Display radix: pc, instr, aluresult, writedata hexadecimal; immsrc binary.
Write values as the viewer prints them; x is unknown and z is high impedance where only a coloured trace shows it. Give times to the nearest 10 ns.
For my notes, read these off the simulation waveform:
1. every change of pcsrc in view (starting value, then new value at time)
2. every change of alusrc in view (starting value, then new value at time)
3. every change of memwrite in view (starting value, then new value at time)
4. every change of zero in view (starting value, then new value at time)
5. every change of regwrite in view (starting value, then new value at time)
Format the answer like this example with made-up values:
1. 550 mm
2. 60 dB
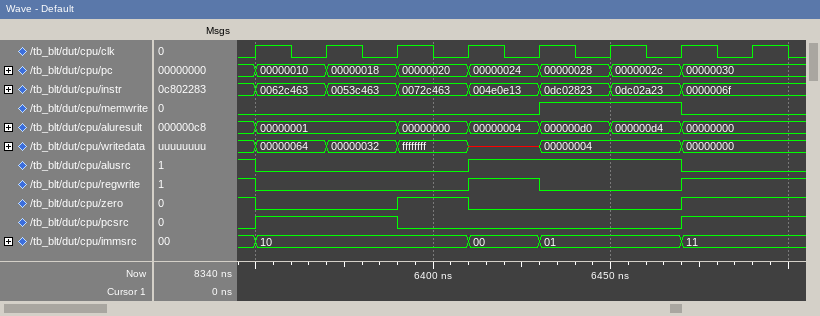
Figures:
1. 0, 1 at 6350 ns, 0 at 6390 ns, 1 at 6470 ns
2. 1, 0 at 6350 ns, 1 at 6410 ns, 0 at 6470 ns
3. 0, 1 at 6430 ns, 0 at 6470 ns
4. 1, 0 at 6350 ns, 1 at 6390 ns, 0 at 6410 ns, 1 at 6470 ns
5. 1, 0 at 6350 ns, 1 at 6410 ns, 0 at 6430 ns, 1 at 6470 ns
